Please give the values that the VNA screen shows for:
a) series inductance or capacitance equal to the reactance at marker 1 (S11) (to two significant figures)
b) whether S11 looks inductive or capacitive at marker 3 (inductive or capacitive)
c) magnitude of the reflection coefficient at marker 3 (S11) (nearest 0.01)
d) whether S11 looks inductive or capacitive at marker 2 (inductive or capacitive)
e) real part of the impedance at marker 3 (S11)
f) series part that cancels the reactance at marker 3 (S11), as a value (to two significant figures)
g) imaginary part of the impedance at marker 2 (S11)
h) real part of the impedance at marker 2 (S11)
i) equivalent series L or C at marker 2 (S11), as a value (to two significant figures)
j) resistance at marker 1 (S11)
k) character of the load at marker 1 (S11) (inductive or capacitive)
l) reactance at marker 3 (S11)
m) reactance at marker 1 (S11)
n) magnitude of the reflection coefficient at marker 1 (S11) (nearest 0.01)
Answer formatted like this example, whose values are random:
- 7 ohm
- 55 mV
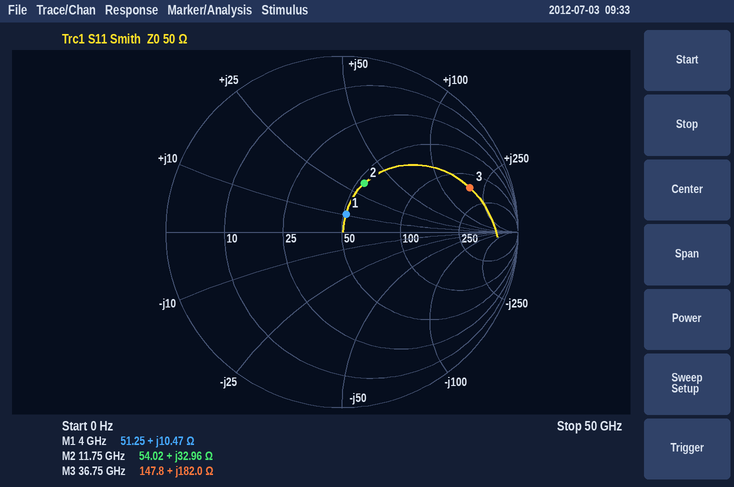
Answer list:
- 420 pH
- inductive
- 0.77
- inductive
- 147.8 Ω
- 24 fF
- +32.96 Ω
- 54.02 Ω
- 450 pH
- 51.25 Ω
- inductive
- +182.0 Ω
- +10.47 Ω
- 0.10
